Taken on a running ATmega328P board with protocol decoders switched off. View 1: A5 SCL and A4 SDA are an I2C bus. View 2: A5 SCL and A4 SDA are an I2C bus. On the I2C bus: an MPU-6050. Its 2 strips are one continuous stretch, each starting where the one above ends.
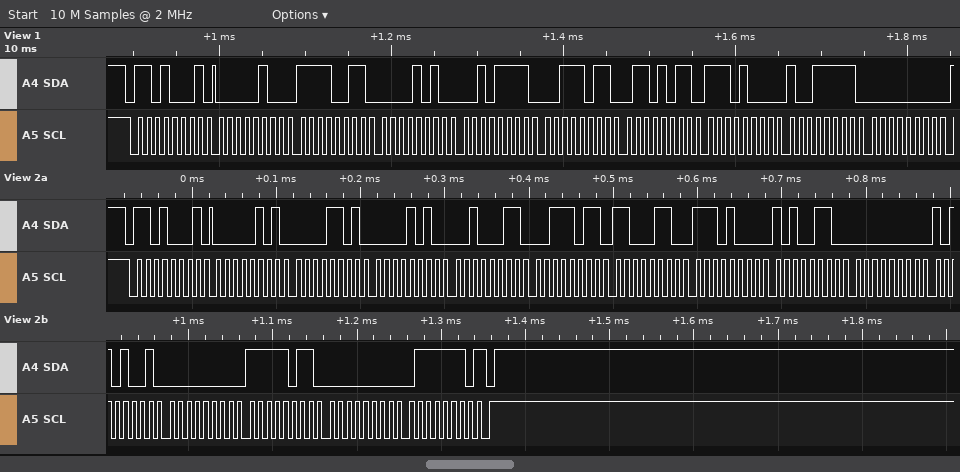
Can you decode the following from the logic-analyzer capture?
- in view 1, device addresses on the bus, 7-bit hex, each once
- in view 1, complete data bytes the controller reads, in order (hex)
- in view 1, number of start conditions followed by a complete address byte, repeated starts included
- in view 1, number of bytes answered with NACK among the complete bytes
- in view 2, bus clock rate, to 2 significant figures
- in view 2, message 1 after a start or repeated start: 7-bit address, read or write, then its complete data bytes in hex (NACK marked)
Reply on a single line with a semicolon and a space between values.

0x68; 04 F3 0A 2F 3B 6B E8 9F 00; 1; 0; 100 kHz; 0x68 read: 05 0D 0A 23 3B C6 E8 A6 00 A9 00 FB 00 7E NACK
